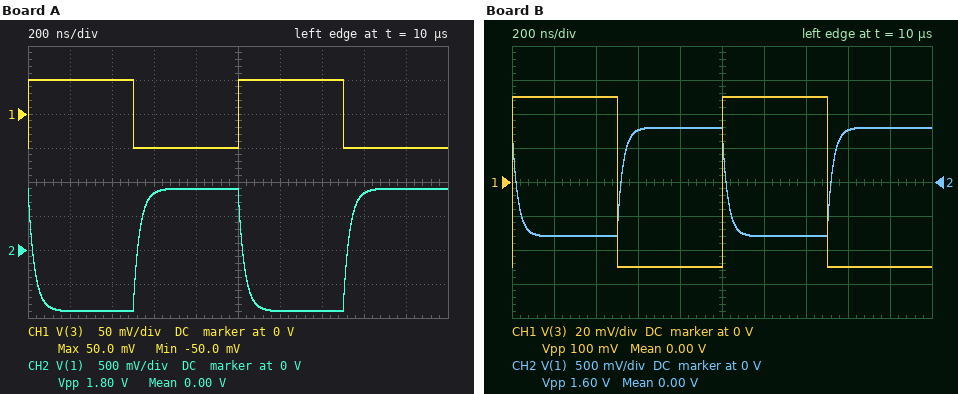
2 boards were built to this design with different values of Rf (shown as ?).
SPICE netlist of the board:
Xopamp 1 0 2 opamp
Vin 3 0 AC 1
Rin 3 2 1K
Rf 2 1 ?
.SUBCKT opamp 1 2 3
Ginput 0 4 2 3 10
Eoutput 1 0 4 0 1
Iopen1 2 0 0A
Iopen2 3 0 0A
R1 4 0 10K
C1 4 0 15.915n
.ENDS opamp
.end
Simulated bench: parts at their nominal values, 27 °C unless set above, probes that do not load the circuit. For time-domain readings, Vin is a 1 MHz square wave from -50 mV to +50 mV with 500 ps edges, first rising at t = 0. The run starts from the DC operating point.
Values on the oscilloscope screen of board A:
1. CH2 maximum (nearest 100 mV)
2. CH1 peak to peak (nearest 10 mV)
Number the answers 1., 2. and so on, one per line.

1. 900 mV
2. 100 mV
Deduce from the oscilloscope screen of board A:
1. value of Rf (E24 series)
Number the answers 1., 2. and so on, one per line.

1. 18 kΩ
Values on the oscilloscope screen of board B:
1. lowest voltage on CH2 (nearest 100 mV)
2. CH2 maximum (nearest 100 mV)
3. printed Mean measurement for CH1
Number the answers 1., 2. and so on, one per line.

1. -800 mV
2. 800 mV
3. 0.00 V
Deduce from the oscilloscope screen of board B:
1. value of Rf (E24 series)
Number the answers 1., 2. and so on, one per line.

1. 16 kΩ
